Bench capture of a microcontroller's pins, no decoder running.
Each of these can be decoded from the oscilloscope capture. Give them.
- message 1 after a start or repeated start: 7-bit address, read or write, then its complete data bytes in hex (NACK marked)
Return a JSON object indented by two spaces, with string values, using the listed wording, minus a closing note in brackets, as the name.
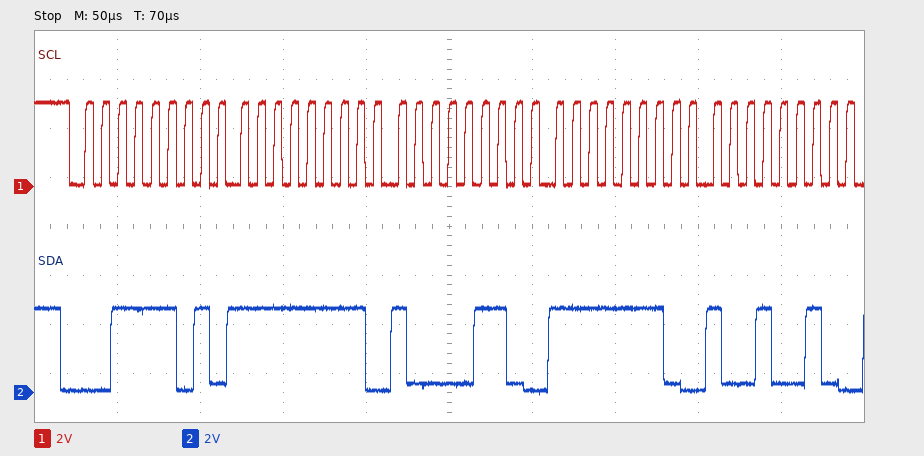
{
  "message 1 after a start or repeated start: 7-bit address, read or write, then its complete data bytes in hex": "0x1E read: FF 86 FE 92"
}
